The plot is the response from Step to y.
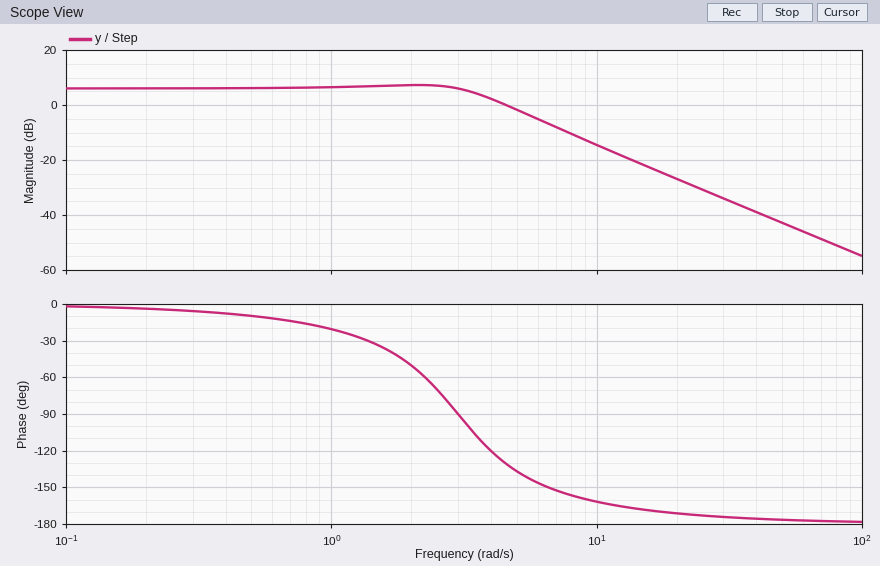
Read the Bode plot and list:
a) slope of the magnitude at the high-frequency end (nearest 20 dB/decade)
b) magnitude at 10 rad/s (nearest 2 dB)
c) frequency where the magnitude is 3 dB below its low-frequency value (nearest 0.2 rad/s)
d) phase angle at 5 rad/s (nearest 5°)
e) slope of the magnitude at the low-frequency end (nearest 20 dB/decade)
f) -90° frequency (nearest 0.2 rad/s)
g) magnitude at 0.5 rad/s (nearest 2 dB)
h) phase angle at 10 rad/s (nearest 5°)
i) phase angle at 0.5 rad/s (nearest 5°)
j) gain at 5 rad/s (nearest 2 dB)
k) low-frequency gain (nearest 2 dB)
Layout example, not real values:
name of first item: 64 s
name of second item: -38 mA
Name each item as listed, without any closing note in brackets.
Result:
slope of the magnitude at the high-frequency end: -40 dB/decade
magnitude at 10 rad/s: -14 dB
frequency where the magnitude is 3 dB below its low-frequency value: 3.8 rad/s
phase angle at 5 rad/s: -135°
slope of the magnitude at the low-frequency end: 0 dB/decade
-90° frequency: 3.0 rad/s
magnitude at 0.5 rad/s: 6 dB
phase angle at 10 rad/s: -160°
phase angle at 0.5 rad/s: -10°
gain at 5 rad/s: -2 dB
low-frequency gain: 6 dB
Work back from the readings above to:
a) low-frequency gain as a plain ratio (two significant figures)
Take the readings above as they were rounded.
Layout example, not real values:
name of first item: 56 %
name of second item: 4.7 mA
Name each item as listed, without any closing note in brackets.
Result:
low-frequency gain as a plain ratio: 2.0
